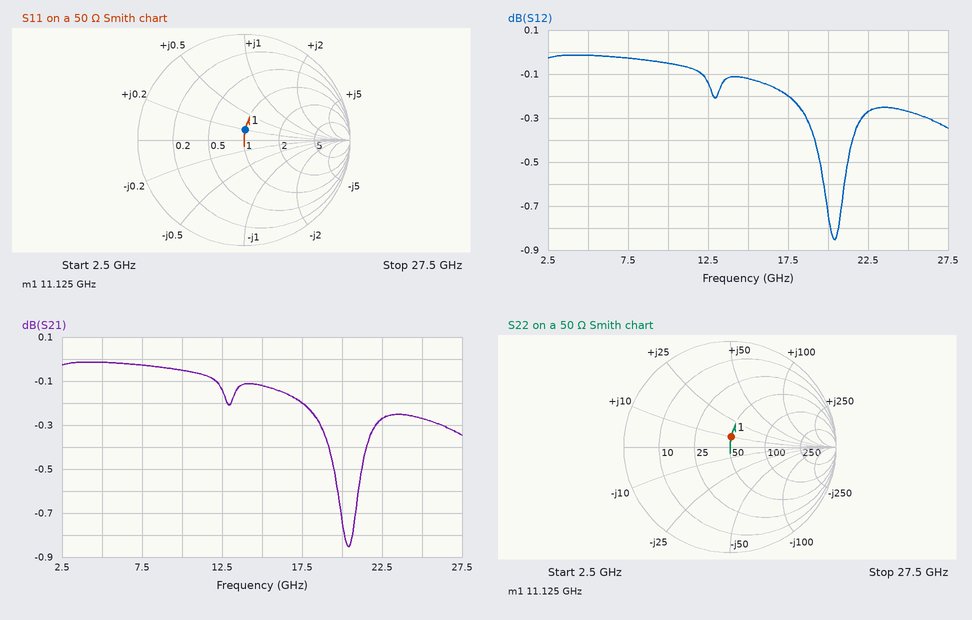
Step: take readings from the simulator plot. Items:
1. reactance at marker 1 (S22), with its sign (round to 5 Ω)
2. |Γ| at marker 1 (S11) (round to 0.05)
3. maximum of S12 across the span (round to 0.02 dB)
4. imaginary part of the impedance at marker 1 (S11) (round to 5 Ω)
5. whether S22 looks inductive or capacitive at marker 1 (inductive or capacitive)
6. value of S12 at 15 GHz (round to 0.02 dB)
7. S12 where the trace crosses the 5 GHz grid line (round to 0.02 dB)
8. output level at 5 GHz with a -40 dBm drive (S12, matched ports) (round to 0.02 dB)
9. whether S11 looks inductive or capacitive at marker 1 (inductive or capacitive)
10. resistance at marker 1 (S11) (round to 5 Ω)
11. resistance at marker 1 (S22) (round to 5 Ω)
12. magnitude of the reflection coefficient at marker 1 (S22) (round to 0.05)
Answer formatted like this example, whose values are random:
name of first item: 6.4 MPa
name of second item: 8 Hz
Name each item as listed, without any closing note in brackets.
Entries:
reactance at marker 1 (S22), with its sign: +10 Ω
|Γ| at marker 1 (S11): 0.10
maximum of S12 across the span: -0.02 dB
imaginary part of the impedance at marker 1 (S11): +10 Ω
whether S22 looks inductive or capacitive at marker 1: inductive
value of S12 at 15 GHz: -0.12 dB
S12 where the trace crosses the 5 GHz grid line: -0.02 dB
output level at 5 GHz with a -40 dBm drive (S12, matched ports): -40.02 dBm
whether S11 looks inductive or capacitive at marker 1: inductive
resistance at marker 1 (S11): 50 Ω
resistance at marker 1 (S22): 50 Ω
magnitude of the reflection coefficient at marker 1 (S22): 0.10
